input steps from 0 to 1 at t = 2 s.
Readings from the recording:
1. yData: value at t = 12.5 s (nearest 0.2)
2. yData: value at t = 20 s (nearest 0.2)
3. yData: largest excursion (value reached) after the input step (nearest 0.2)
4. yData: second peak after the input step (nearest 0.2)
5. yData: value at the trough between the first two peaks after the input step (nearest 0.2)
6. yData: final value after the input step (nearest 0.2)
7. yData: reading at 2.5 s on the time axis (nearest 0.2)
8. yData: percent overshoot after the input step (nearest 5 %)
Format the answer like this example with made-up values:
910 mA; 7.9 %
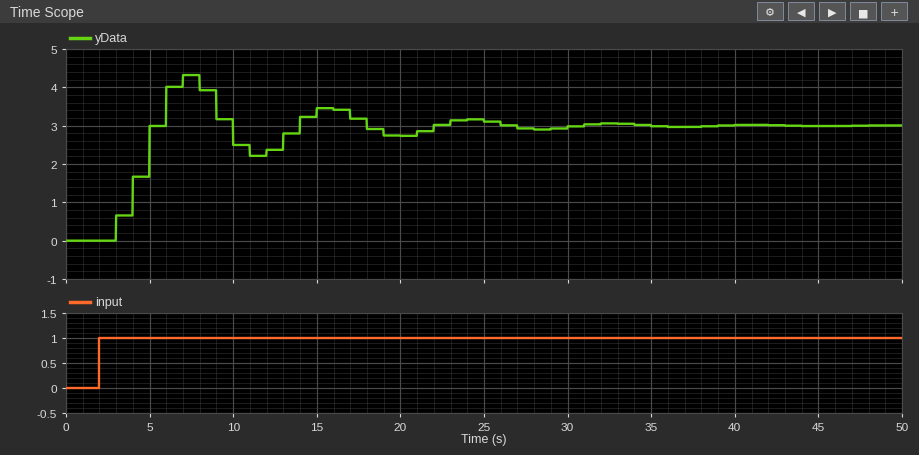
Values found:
2.4; 2.8; 4.4; 3.4; 2.2; 3.0; 0.0; 45 %
